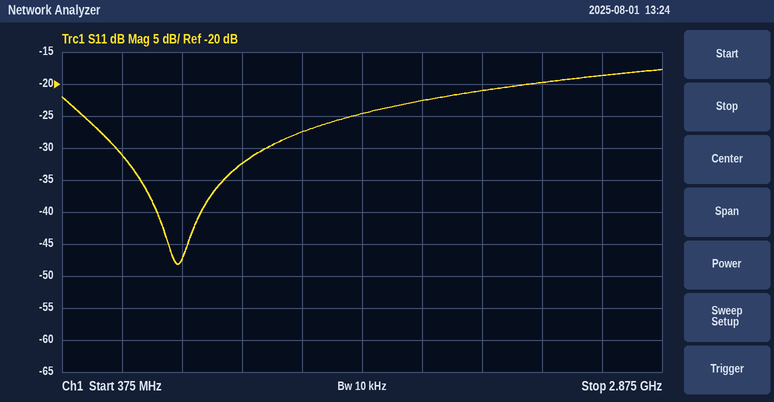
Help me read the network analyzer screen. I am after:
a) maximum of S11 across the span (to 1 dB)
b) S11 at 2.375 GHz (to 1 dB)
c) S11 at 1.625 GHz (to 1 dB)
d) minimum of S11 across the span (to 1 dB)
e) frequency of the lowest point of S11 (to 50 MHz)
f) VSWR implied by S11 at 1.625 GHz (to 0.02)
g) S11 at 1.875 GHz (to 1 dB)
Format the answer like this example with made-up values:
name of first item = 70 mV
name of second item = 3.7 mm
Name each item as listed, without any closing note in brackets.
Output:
maximum of S11 across the span = -18 dB
S11 at 2.375 GHz = -20 dB
S11 at 1.625 GHz = -25 dB
minimum of S11 across the span = -48 dB
frequency of the lowest point of S11 = 850 MHz
VSWR implied by S11 at 1.625 GHz = 1.12
S11 at 1.875 GHz = -23 dB
